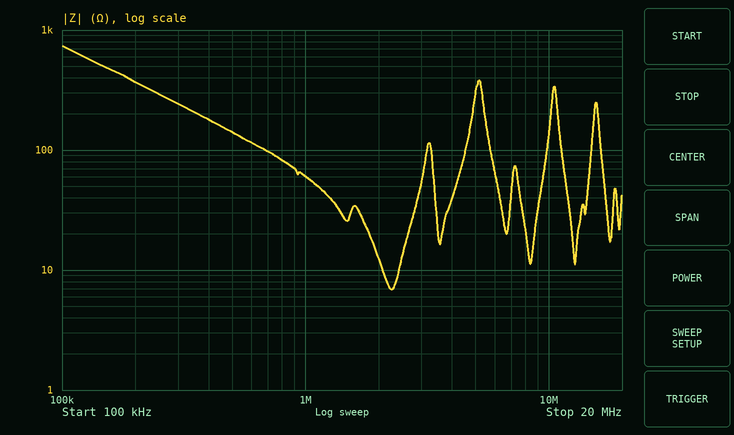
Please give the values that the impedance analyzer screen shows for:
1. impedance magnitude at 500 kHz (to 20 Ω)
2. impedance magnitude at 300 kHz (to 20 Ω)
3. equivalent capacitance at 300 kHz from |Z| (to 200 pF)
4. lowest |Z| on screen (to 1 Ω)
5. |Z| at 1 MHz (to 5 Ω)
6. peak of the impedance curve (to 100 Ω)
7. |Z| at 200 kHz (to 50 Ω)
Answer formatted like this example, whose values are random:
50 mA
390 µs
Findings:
140 Ω
240 Ω
2.2 nF
7 Ω
60 Ω
700 Ω
350 Ω
